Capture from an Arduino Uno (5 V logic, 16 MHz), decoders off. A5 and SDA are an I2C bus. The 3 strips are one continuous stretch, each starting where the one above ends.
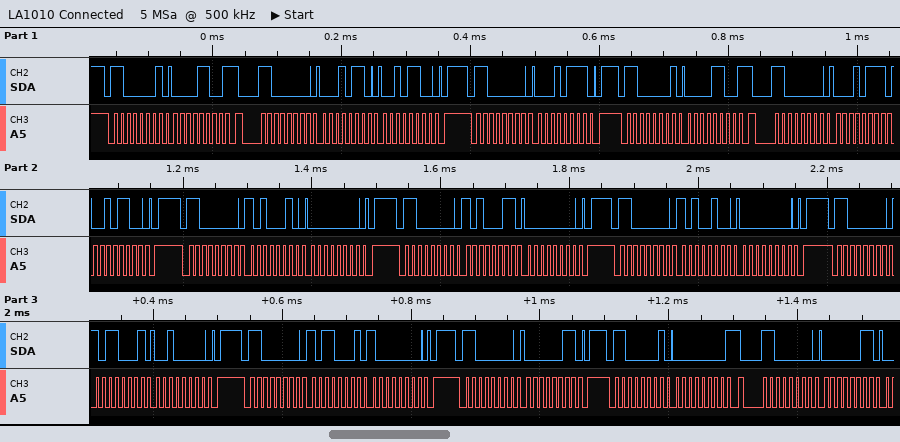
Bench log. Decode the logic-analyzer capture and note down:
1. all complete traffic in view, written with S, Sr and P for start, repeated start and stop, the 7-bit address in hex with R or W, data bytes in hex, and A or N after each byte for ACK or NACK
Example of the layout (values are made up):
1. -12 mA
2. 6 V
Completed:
1. S 60R A 0C N Sr 60W A 16 A 2C A P S 60W A 17 A P S 60R A 0C N Sr 60W A 17 A 2C A P S 60W A A2 A 00 A P S 60W A A3 A 00 A P S 60W A A4 A 00 A P S 60W A B1 A 20 A P S 60W A B1 A 80 A P S 60W A 03 A P S 60R A 00 N Sr 60W A 03 A
